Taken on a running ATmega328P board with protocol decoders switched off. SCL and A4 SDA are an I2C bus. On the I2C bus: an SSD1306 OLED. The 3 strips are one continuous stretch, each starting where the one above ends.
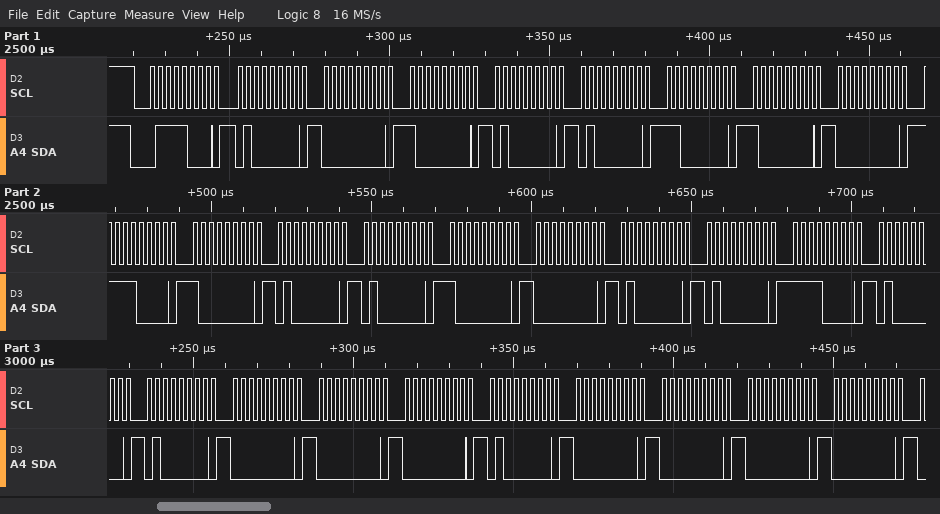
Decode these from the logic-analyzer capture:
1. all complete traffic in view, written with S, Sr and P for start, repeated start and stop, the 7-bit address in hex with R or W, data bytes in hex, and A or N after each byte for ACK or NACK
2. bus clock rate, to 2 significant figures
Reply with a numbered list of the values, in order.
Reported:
1. S 3CW A 40 A 00 A 80 A 40 A 40 A C0 A 80 A 00 A F0 A 80 A 40 A 40 A 80 A 00 A 40 A 40 A F0 A 40 A 40 A 00 A 00 A 00 A 40 A 00 A 00 A 00 A 00 A
2. 400 kHz
